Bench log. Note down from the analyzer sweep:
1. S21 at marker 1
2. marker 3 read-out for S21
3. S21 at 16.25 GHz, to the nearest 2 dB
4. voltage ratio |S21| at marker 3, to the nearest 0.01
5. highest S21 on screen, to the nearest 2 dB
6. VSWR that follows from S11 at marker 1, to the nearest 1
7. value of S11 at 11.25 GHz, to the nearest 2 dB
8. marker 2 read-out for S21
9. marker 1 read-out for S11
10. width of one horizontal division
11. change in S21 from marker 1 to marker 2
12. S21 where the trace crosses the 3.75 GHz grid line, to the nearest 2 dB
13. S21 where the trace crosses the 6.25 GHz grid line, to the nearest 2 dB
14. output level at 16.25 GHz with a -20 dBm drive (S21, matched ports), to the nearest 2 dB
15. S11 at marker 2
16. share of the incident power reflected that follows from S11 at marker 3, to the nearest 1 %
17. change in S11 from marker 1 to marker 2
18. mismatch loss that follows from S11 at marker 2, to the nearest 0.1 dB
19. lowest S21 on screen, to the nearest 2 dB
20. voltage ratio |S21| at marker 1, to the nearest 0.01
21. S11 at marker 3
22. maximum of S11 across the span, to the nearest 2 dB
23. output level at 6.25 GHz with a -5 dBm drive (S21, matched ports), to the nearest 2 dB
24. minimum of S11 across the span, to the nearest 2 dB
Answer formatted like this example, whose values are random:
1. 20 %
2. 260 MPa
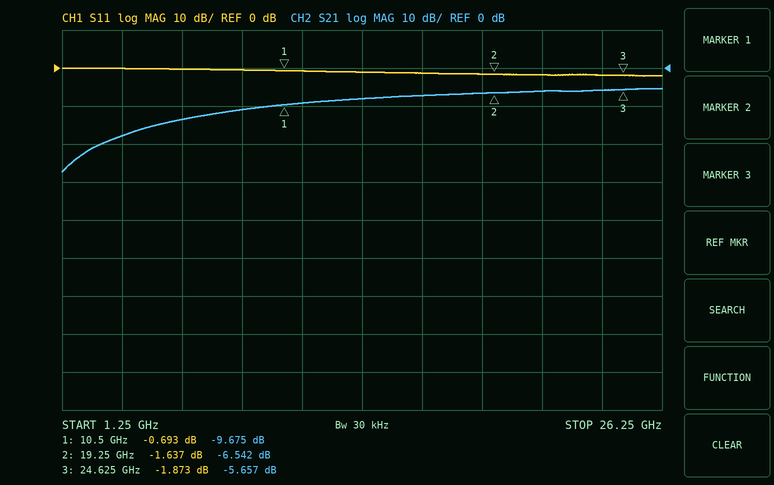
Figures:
1. -9.675 dB
2. -5.657 dB
3. -8 dB
4. 0.52
5. -6 dB
6. 25
7. 0 dB
8. -6.542 dB
9. -0.693 dB
10. 2.5 GHz
11. 3.133 dB
12. -18 dB
13. -14 dB
14. -28 dBm
15. -1.637 dB
16. 65 %
17. -0.944 dB
18. 5.0 dB
19. -28 dB
20. 0.33
21. -1.873 dB
22. 0 dB
23. -18 dBm
24. -2 dB
